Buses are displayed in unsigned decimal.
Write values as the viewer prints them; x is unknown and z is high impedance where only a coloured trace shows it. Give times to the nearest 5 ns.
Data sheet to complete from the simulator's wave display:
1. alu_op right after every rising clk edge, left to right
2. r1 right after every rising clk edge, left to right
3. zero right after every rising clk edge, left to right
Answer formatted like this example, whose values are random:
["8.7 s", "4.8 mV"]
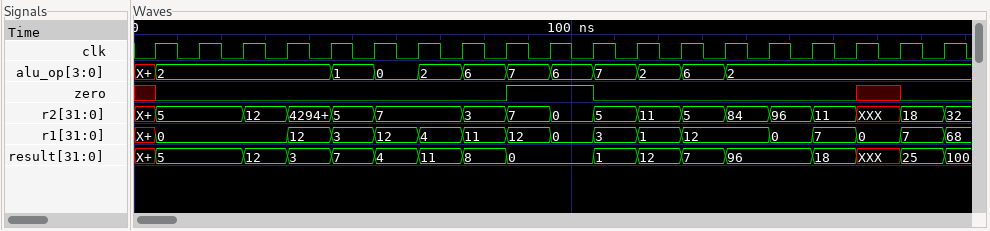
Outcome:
["2, 2, 2, 2, 1, 0, 2, 6, 7, 6, 7, 2, 6, 2, 2, 2, 2, 2, 2", "0, 0, 0, 12, 3, 12, 4, 11, 12, 0, 3, 1, 12, 12, 0, 7, 0, 7, 68", "0 0 0 0 0 0 0 0 1 1 0 0 0 0 0 0 x 0 0"]
